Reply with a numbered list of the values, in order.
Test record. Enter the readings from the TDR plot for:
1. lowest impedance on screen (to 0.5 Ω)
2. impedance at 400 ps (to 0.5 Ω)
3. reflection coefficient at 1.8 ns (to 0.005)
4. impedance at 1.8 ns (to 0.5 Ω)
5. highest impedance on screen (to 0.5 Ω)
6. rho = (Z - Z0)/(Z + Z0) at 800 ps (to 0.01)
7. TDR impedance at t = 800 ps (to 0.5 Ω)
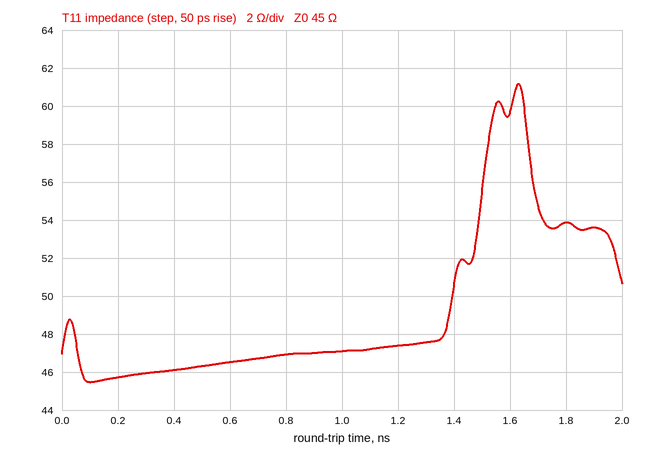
1. 45.5 Ω
2. 46.0 Ω
3. +0.090
4. 54.0 Ω
5. 61.0 Ω
6. +0.02
7. 47.0 Ω
